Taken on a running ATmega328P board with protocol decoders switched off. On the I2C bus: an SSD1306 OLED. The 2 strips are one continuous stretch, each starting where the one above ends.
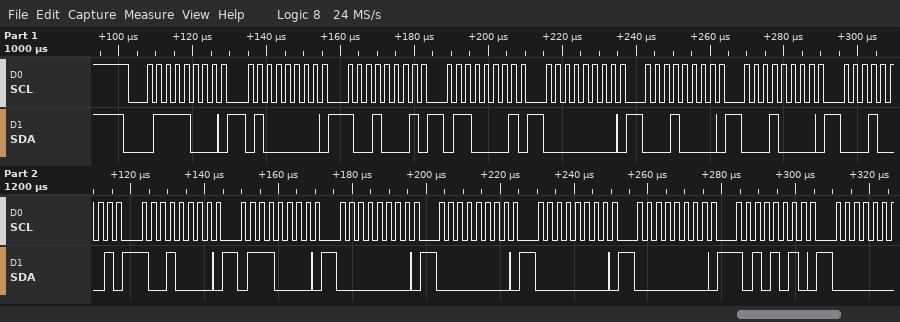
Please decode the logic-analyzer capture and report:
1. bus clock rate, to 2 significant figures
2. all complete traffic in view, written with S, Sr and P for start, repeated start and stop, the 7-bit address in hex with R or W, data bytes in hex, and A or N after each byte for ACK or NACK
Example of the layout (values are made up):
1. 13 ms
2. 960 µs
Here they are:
1. 400 kHz
2. S 3CW A 40 A 91 A 61 A 00 A 10 A 10 A 11 A 90 A 70 A 00 A 00 A 00 A 00 A AA A
